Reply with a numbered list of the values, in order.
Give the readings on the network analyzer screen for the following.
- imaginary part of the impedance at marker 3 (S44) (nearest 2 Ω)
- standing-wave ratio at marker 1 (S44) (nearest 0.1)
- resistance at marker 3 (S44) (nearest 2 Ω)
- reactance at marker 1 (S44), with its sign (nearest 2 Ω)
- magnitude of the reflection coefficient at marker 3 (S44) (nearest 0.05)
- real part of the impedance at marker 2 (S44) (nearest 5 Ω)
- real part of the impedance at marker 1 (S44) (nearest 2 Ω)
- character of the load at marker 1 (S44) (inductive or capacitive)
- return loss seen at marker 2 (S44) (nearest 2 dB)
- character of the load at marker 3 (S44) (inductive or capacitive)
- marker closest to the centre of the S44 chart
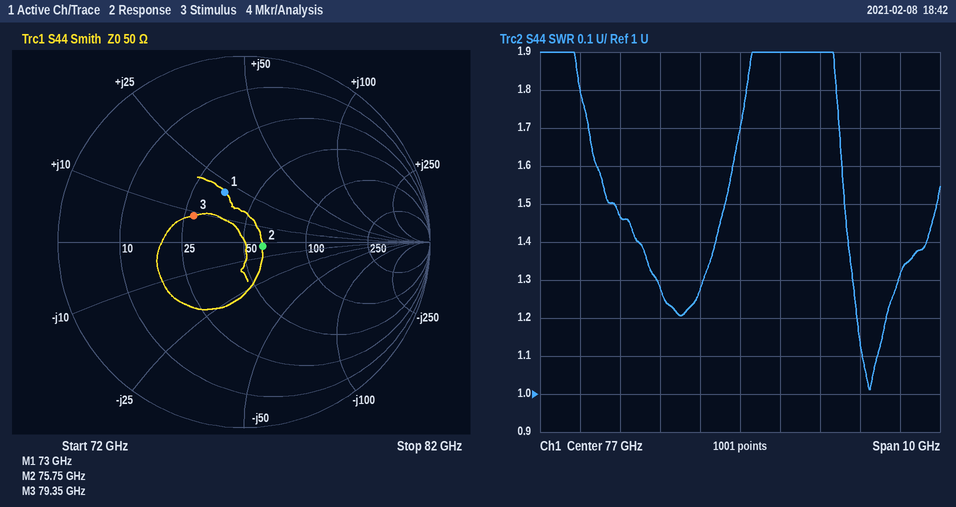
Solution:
1. +8 Ω
2. 1.8
3. 28 Ω
4. +20 Ω
5. 0.30
6. 60 Ω
7. 36 Ω
8. inductive
9. 20 dB
10. inductive
11. marker 2
